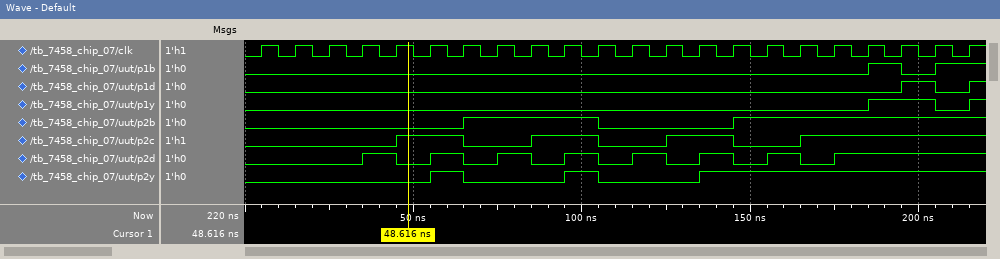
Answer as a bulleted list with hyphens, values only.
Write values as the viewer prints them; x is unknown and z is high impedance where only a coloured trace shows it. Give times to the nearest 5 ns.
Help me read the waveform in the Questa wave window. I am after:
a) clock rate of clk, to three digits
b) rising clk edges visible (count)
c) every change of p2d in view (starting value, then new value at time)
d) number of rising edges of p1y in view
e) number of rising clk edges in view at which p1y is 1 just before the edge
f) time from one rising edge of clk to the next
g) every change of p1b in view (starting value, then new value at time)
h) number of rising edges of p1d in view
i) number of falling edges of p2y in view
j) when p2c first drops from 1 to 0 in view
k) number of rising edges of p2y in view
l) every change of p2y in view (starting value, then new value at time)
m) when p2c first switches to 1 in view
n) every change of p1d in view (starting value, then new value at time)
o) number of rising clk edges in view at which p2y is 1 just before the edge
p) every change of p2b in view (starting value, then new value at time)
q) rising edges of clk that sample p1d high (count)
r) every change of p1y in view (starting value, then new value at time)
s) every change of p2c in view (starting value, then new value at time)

- 100 MHz
- 22
- 0, 1 at 35 ns, 0 at 45 ns, 1 at 55 ns, 0 at 65 ns, 1 at 75 ns, 0 at 85 ns, 1 at 95 ns, 0 at 105 ns, 1 at 115 ns, 0 at 125 ns, 1 at 135 ns, 0 at 145 ns, 1 at 155 ns, 0 at 165 ns, 1 at 175 ns
- 2
- 2
- 10 ns
- 0, 1 at 185 ns, 0 at 195 ns, 1 at 205 ns
- 2
- 2
- 65 ns
- 3
- 0, 1 at 55 ns, 0 at 65 ns, 1 at 95 ns, 0 at 105 ns, 1 at 135 ns
- 45 ns
- 0, 1 at 195 ns, 0 at 205 ns, 1 at 215 ns
- 10
- 0, 1 at 65 ns, 0 at 105 ns, 1 at 145 ns
- 1
- 0, 1 at 185 ns, 0 at 205 ns, 1 at 215 ns
- 0, 1 at 45 ns, 0 at 65 ns, 1 at 85 ns, 0 at 105 ns, 1 at 125 ns, 0 at 145 ns, 1 at 165 ns
